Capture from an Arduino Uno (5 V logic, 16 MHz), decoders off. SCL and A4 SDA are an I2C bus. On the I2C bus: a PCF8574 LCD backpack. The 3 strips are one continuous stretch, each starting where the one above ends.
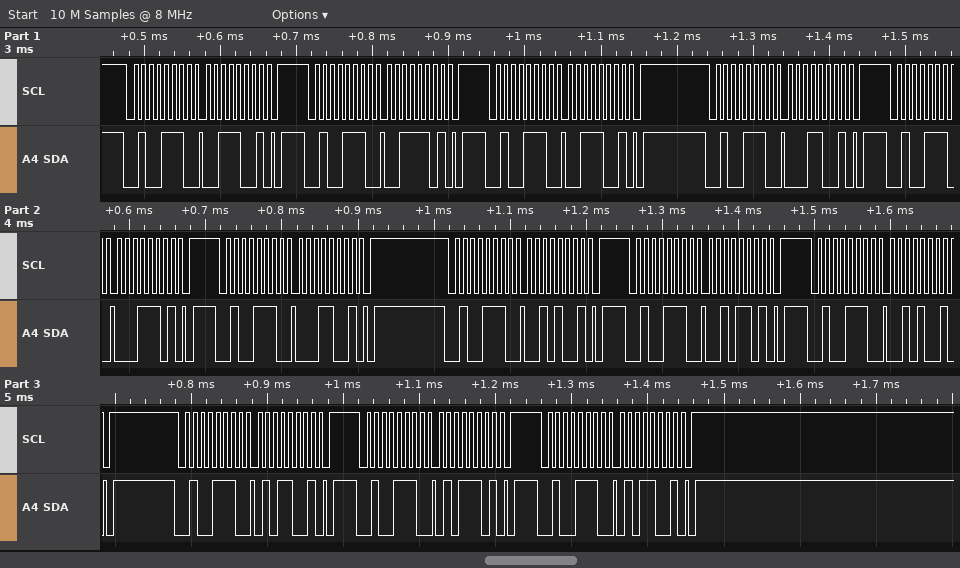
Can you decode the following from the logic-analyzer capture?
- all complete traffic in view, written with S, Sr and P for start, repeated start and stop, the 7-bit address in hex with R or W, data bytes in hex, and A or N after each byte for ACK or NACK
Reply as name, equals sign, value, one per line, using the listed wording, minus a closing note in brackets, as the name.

all complete traffic in view, written with S, Sr and P for start, repeated start and stop, the 7-bit address in hex with R or W, data bytes in hex, and A or N after each byte for ACK or NACK = S 27W A 39 A P S 27W A 3D A P S 27W A 39 A P S 27W A 19 A P S 27W A 1D A P S 27W A 19 A P S 27W A 29 A P S 27W A 2D A P S 27W A 29 A P S 27W A 59 A P S 27W A 5D A P S 27W A 59 A P
